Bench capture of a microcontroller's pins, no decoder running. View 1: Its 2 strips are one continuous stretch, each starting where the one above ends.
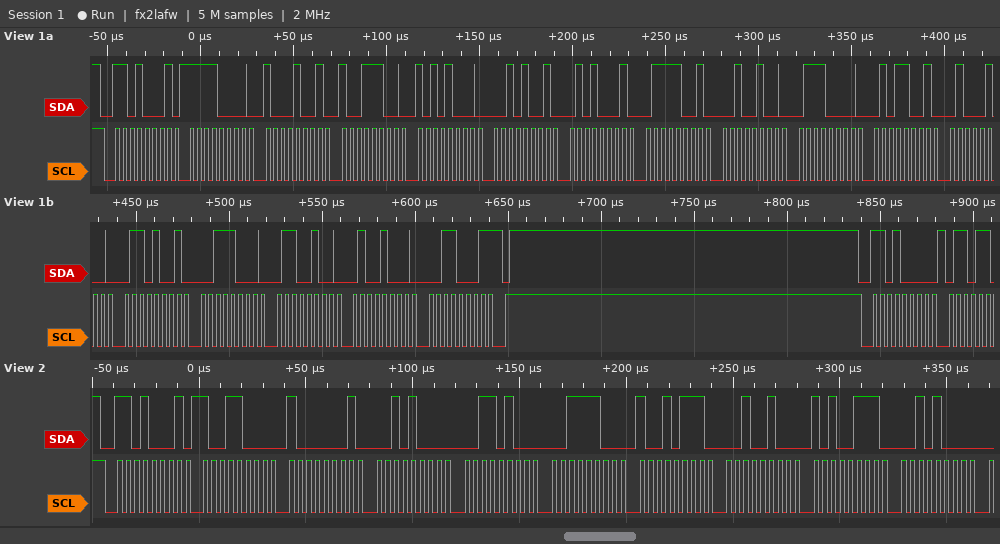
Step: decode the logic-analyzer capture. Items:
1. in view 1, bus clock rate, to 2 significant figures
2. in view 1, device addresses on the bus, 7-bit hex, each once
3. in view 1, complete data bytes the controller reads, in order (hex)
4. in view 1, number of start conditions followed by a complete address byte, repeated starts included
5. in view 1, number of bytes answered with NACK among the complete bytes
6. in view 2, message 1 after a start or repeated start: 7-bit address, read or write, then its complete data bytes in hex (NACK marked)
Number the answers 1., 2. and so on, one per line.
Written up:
1. 250 kHz
2. 0x68
3. F0 89 9C A8 29 51 79 24 70 59 44 69 38 64 48 31
4. 2
5. 1
6. 0x68 read: 98 81 28 34 3C 97 24 A7 28
